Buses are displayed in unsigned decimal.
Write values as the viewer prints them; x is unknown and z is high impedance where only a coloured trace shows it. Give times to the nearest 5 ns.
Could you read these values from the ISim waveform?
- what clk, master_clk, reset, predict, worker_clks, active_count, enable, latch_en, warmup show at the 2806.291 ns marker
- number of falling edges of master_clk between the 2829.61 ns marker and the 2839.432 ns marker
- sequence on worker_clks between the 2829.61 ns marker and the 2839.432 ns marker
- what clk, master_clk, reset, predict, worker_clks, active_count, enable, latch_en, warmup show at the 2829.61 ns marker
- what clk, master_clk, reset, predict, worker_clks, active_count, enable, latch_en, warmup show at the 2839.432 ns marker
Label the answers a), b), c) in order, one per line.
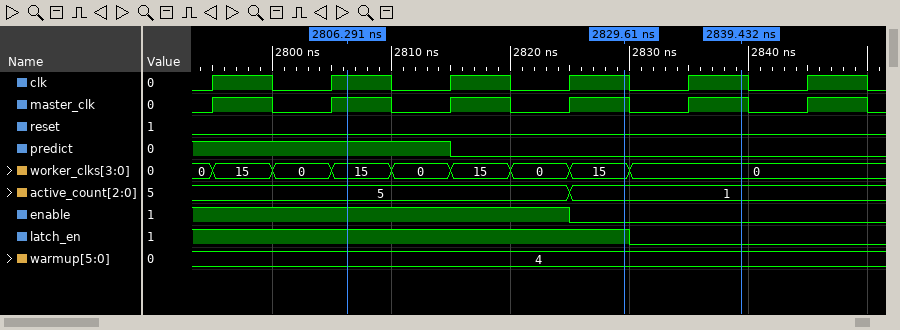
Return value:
a) clk=1, master_clk=1, reset=0, predict=1, worker_clks=15, active_count=5, enable=1, latch_en=1, warmup=4
b) 1
c) 15, 0
d) clk=1, master_clk=1, reset=0, predict=0, worker_clks=15, active_count=1, enable=0, latch_en=1, warmup=4
e) clk=1, master_clk=1, reset=0, predict=0, worker_clks=0, active_count=1, enable=0, latch_en=0, warmup=4
